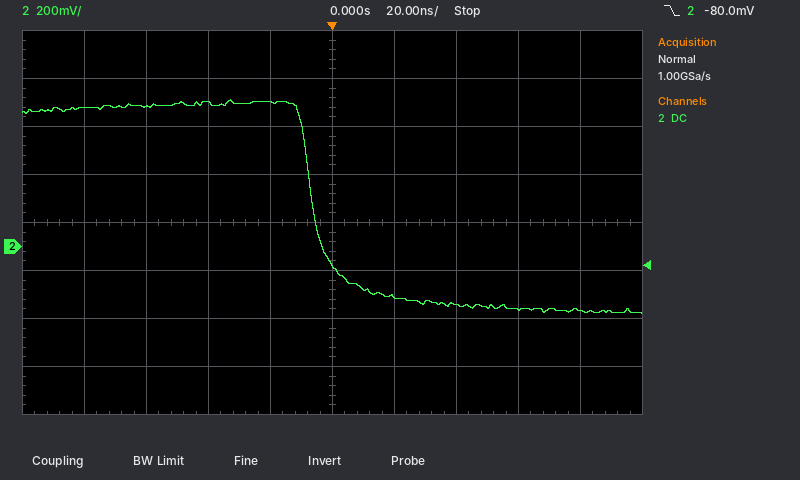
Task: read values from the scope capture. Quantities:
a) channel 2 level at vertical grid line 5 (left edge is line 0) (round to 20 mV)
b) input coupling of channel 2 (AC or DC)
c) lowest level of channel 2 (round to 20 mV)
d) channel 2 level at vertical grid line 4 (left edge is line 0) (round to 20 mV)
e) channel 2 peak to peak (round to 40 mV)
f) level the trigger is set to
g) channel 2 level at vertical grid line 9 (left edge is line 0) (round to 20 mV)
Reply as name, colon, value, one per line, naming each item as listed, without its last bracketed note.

channel 2 level at vertical grid line 5 (left edge is line 0): -80 mV
input coupling of channel 2: DC
lowest level of channel 2: -280 mV
channel 2 level at vertical grid line 4 (left edge is line 0): 600 mV
channel 2 peak to peak: 880 mV
level the trigger is set to: -80.0 mV
channel 2 level at vertical grid line 9 (left edge is line 0): -260 mV
